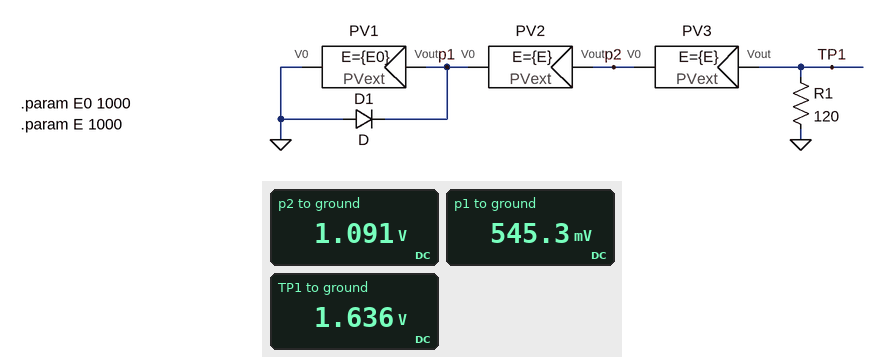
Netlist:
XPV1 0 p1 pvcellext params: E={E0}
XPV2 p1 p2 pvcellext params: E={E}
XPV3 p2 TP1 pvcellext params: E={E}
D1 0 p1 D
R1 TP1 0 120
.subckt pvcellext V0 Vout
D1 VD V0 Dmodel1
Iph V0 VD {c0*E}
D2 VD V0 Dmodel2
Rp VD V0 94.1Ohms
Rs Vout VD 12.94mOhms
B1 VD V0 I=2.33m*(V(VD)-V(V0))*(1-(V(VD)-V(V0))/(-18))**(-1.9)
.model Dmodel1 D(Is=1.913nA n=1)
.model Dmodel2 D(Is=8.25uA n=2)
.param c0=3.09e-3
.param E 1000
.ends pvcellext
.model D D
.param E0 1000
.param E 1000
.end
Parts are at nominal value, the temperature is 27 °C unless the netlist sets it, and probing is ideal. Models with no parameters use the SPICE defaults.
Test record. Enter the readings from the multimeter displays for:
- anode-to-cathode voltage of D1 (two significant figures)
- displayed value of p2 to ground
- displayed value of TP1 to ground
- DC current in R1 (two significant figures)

-550 mV
1.091 V
1.636 V
14 mA
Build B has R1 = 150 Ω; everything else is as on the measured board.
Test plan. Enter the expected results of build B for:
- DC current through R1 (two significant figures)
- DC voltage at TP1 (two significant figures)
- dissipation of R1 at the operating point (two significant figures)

11 mA
1.6 V
18 mW
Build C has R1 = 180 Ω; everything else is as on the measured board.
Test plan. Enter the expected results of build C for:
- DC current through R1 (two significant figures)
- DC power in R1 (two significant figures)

9.1 mA
15 mW
